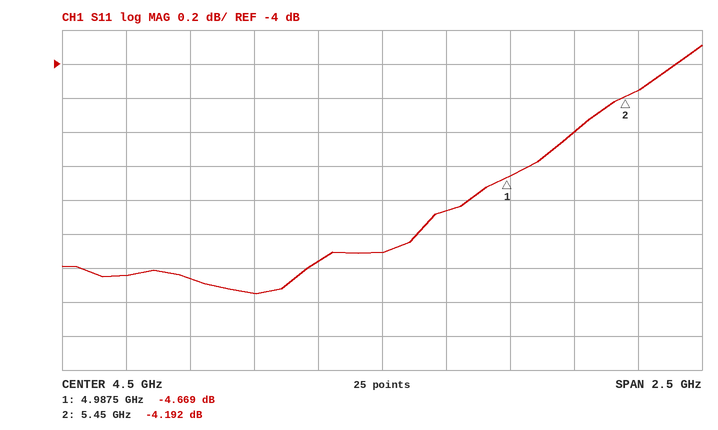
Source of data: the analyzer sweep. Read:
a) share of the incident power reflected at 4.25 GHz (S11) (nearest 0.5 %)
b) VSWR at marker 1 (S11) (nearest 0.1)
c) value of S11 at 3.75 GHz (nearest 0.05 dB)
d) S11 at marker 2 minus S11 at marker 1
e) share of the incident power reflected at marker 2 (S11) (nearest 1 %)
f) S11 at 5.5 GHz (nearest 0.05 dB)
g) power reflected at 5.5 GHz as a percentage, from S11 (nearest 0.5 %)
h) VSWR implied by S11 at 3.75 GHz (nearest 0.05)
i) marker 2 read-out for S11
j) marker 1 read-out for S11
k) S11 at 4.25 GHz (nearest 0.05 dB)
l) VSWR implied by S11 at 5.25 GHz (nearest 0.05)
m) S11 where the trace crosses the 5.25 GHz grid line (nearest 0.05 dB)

30.5 %
3.8
-5.25 dB
0.477 dB
38 %
-4.15 dB
38.5 %
3.40
-4.192 dB
-4.669 dB
-5.15 dB
4.05
-4.40 dB
